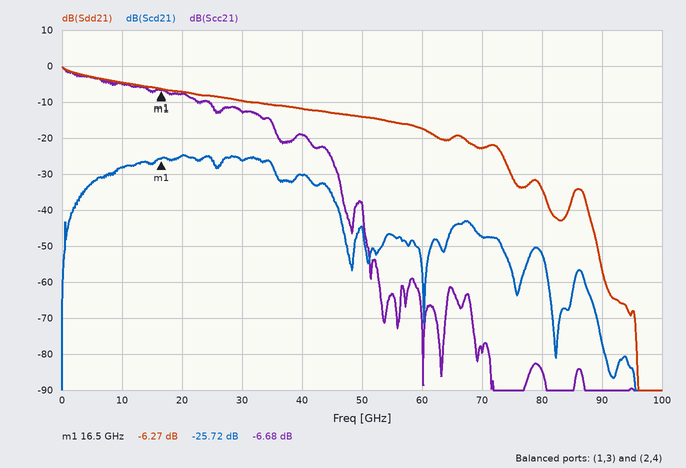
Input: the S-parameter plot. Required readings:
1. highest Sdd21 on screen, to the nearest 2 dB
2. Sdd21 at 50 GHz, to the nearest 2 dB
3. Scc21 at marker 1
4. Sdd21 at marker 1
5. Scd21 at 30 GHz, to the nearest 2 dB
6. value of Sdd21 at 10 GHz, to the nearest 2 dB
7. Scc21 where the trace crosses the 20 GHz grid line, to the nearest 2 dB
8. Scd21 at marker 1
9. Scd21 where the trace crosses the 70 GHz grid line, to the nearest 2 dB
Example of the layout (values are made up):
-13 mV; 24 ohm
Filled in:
0 dB; -14 dB; -6.68 dB; -6.27 dB; -26 dB; -4 dB; -8 dB; -25.72 dB; -48 dB
